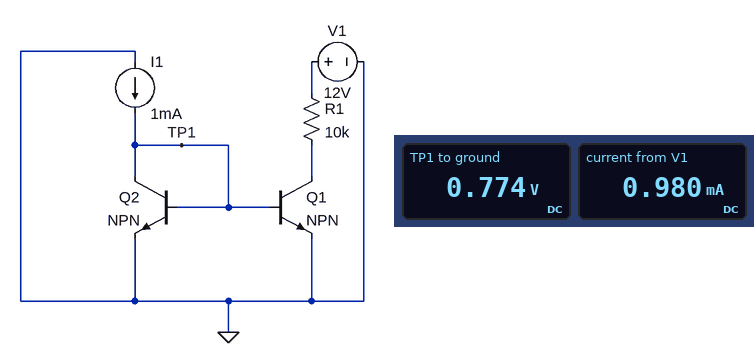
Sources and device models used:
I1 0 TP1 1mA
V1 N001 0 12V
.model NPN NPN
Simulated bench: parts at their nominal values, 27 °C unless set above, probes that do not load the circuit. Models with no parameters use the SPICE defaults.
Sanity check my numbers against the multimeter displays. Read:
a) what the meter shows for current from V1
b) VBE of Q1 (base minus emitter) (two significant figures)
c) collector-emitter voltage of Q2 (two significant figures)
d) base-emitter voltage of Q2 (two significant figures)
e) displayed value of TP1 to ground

0.980 mA
770 mV
770 mV
770 mV
0.774 V
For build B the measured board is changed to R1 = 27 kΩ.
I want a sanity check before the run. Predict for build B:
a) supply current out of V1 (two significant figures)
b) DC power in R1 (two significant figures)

440 µA
5.3 mW
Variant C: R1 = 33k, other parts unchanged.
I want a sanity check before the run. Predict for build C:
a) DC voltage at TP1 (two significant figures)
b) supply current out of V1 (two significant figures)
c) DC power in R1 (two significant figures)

770 mV
360 µA
4.3 mW
